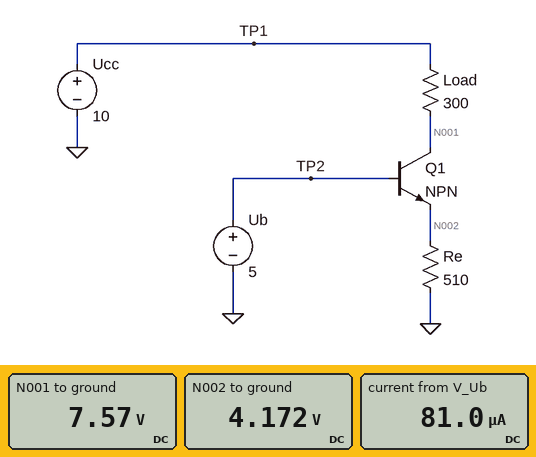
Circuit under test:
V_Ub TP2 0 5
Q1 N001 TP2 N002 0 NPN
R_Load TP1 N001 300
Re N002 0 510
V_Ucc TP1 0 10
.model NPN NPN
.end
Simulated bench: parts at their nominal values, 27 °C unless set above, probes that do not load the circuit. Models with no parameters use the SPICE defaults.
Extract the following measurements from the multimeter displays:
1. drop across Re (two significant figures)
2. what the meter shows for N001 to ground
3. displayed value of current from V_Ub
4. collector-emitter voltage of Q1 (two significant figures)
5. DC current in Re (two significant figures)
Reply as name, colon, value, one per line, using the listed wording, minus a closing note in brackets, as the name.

drop across Re: 4.2 V
what the meter shows for N001 to ground: 7.57 V
displayed value of current from V_Ub: 81.0 µA
collector-emitter voltage of Q1: 3.4 V
DC current in Re: 8.2 mA
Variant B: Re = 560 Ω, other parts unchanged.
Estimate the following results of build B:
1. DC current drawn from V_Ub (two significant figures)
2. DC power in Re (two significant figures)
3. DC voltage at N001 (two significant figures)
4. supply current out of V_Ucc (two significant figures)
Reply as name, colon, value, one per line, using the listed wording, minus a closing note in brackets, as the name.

DC current drawn from V_Ub: 74 µA
DC power in Re: 31 mW
DC voltage at N001: 7.8 V
supply current out of V_Ucc: 7.4 mA
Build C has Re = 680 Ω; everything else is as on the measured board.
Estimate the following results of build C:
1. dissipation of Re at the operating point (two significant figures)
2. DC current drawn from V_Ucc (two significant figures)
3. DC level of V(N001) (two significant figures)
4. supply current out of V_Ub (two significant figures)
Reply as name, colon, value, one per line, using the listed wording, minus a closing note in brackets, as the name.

dissipation of Re at the operating point: 26 mW
DC current drawn from V_Ucc: 6.1 mA
DC level of V(N001): 8.2 V
supply current out of V_Ub: 61 µA
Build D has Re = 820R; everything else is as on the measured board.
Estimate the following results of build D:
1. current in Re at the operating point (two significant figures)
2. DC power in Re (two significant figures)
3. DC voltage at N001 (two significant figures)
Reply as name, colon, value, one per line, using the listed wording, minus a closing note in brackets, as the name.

current in Re at the operating point: 5.1 mA
DC power in Re: 21 mW
DC voltage at N001: 8.5 V
